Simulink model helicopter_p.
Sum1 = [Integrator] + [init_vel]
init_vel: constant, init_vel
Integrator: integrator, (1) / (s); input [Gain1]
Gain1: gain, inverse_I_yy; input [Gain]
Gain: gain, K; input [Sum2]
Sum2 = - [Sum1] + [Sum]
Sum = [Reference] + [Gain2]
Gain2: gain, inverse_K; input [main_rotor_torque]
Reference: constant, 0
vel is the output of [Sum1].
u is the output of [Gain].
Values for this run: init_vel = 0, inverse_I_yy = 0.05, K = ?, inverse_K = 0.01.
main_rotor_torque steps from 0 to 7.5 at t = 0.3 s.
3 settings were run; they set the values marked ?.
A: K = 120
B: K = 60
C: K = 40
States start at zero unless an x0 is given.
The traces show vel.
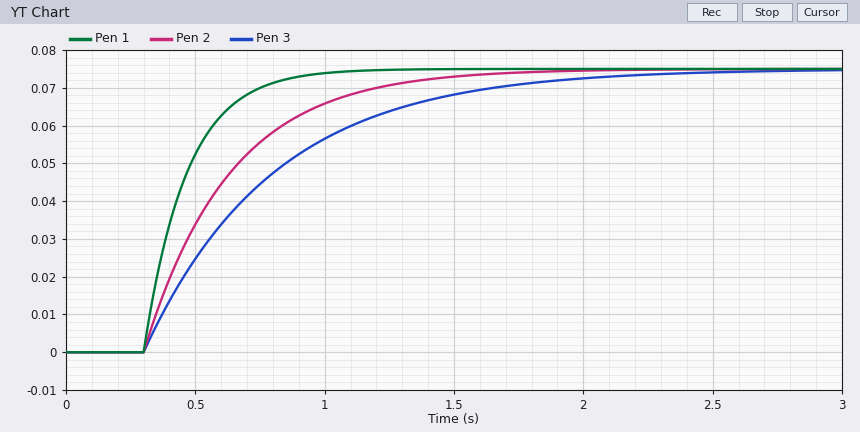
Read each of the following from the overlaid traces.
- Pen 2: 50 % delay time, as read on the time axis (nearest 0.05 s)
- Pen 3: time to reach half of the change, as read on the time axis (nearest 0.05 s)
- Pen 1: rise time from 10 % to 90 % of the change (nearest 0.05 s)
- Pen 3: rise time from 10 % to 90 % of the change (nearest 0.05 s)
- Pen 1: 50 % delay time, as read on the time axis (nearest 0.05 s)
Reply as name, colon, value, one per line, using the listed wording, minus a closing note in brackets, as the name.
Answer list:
Pen 2: 50 % delay time, as read on the time axis: 0.55 s
Pen 3: time to reach half of the change, as read on the time axis: 0.65 s
Pen 1: rise time from 10 % to 90 % of the change: 0.35 s
Pen 3: rise time from 10 % to 90 % of the change: 1.10 s
Pen 1: 50 % delay time, as read on the time axis: 0.40 s
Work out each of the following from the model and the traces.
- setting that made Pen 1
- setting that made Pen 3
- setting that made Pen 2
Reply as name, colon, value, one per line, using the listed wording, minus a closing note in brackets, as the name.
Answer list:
setting that made Pen 1: A
setting that made Pen 3: C
setting that made Pen 2: B
